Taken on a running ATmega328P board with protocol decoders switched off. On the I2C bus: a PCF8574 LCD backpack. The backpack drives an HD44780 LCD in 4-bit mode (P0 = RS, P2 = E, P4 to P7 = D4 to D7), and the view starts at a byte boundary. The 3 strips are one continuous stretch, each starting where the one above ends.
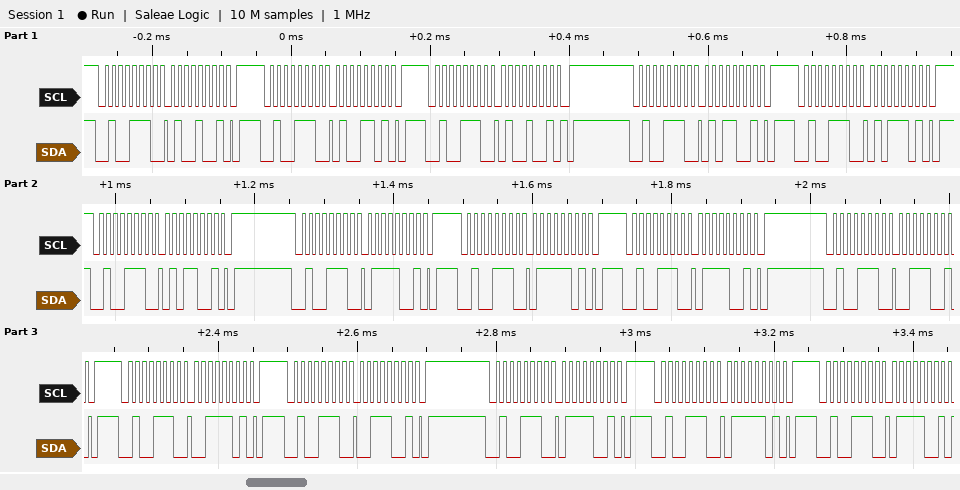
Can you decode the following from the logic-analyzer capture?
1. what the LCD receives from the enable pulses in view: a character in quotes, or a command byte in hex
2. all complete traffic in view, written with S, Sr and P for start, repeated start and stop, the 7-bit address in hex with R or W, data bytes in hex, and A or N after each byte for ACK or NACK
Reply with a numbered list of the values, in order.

1. 'E' 's'
2. S 27W A 49 A P S 27W A 4D A P S 27W A 49 A P S 27W A 59 A P S 27W A 5D A P S 27W A 59 A P S 27W A 79 A P S 27W A 7D A P S 27W A 79 A P S 27W A 39 A P S 27W A 3D A P S 27W A 39 A P S 27W A 79 A P S 27W A 7D A P S 27W A 79 A
